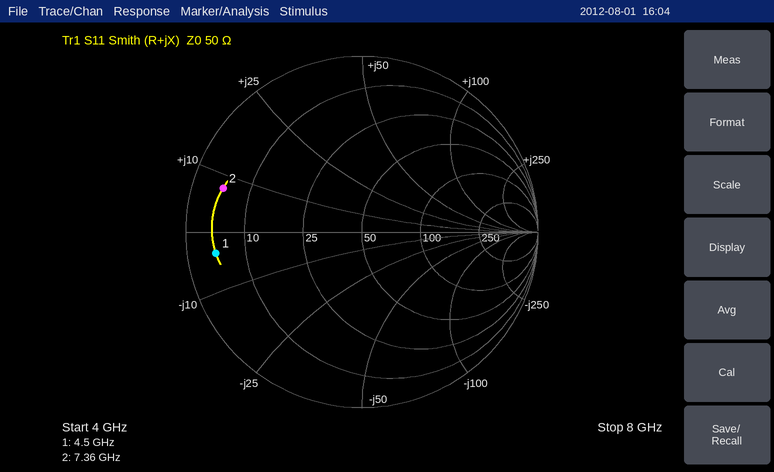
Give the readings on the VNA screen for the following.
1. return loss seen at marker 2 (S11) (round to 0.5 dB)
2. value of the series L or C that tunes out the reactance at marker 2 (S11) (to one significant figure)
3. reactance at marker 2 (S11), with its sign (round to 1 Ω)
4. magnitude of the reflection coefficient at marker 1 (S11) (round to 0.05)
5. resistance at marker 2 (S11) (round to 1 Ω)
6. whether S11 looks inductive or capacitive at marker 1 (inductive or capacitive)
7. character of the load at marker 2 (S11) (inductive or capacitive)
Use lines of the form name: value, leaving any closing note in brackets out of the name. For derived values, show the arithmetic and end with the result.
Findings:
return loss seen at marker 2 (S11): 1.5 dB
value of the series L or C that tunes out the reactance at marker 2 (S11): C = 1/(2π × 7.36 GHz × 8 Ω) ≈ 3 pF
reactance at marker 2 (S11), with its sign: +8 Ω
magnitude of the reflection coefficient at marker 1 (S11): 0.85
resistance at marker 2 (S11): 5 Ω
whether S11 looks inductive or capacitive at marker 1: capacitive
character of the load at marker 2 (S11): inductive
